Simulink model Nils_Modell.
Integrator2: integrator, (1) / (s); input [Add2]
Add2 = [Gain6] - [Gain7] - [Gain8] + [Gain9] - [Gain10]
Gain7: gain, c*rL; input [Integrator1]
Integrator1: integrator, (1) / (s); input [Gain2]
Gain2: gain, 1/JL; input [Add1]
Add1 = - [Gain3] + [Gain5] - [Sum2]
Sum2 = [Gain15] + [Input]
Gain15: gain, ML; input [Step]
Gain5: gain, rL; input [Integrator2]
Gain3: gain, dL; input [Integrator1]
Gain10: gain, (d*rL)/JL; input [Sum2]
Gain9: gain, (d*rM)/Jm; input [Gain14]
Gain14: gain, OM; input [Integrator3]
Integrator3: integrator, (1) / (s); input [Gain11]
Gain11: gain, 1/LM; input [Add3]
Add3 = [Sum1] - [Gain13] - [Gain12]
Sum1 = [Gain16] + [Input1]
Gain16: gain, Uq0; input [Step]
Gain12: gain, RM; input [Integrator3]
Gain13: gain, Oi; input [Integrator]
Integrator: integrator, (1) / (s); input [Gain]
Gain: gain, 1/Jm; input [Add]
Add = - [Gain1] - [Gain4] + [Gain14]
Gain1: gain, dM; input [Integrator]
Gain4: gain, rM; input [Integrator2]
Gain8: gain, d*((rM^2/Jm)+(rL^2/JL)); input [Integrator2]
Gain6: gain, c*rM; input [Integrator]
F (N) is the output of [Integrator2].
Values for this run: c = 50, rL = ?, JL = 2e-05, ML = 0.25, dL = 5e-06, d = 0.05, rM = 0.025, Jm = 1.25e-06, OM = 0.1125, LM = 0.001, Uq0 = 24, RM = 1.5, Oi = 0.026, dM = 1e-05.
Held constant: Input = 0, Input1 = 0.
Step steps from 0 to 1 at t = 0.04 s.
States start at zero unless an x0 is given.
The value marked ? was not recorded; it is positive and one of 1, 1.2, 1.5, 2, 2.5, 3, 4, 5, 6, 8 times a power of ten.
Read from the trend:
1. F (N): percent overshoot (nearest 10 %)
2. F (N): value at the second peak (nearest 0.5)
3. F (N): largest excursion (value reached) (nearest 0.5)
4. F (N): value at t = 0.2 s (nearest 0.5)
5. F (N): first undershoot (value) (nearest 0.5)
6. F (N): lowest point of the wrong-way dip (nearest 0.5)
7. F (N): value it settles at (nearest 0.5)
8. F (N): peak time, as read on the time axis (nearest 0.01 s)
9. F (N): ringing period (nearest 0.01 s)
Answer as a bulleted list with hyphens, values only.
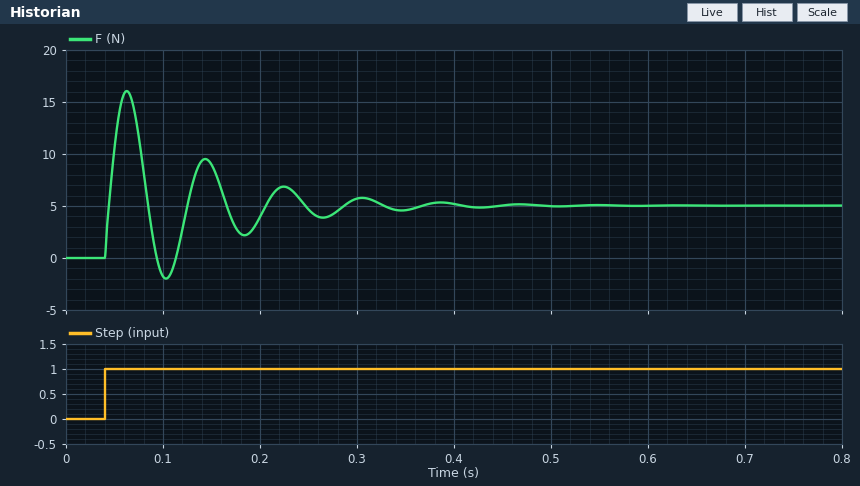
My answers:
- 220 %
- 9.5
- 16.0
- 4.0
- -2.0
- -2.0
- 5.0
- 0.06 s
- 0.08 s
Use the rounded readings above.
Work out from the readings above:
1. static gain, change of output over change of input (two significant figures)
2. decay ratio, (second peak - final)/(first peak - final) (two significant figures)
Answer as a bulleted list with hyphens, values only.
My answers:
- 5.0
- 0.41
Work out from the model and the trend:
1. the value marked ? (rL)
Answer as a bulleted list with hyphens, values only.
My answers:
- 0.05
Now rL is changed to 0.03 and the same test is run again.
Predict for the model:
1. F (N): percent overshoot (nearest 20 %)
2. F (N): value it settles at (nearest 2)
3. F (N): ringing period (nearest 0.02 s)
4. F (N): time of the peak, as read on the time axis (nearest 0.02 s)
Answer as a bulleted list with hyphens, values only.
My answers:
- 200 %
- 8
- 0.14 s
- 0.08 s
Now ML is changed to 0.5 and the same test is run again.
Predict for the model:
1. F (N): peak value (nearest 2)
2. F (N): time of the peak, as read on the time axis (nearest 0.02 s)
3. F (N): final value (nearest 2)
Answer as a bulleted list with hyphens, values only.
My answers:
- 22
- 0.06 s
- 10
